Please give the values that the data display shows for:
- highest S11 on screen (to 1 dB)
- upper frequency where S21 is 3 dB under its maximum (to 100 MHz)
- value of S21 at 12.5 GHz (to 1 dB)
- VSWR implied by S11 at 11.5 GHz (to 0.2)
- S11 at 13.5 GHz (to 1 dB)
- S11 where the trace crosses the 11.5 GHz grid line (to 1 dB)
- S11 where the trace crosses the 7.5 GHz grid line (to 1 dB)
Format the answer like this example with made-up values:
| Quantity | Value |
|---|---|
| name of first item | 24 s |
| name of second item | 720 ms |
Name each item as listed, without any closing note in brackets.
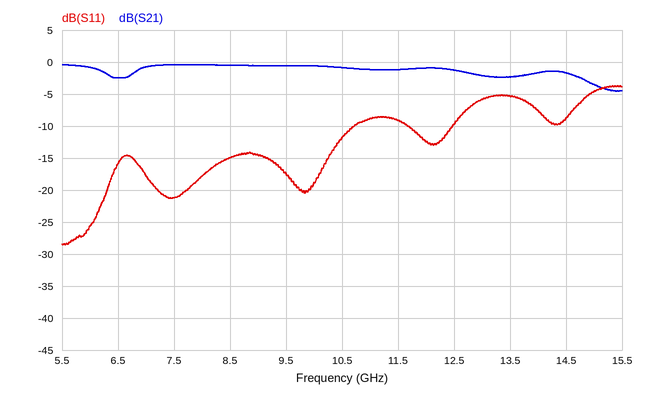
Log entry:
| Quantity | Value |
|---|---|
| highest S11 on screen | -4 dB |
| upper frequency where S21 is 3 dB under its maximum | 15.0 GHz |
| value of S21 at 12.5 GHz | -1 dB |
| VSWR implied by S11 at 11.5 GHz | 2.0 |
| S11 at 13.5 GHz | -5 dB |
| S11 where the trace crosses the 11.5 GHz grid line | -9 dB |
| S11 where the trace crosses the 7.5 GHz grid line | -21 dB |
